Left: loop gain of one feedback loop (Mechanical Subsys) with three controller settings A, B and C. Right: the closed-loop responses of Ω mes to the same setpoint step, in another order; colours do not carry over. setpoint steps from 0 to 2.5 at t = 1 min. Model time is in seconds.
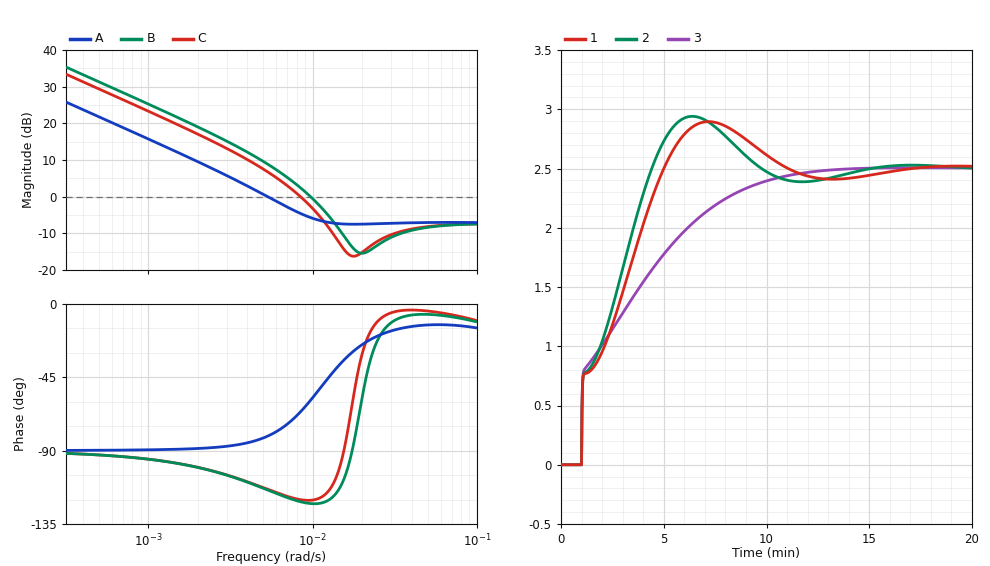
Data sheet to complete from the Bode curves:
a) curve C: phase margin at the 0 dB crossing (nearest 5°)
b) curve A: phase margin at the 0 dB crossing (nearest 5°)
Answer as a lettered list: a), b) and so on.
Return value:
a) 60°
b) 100°
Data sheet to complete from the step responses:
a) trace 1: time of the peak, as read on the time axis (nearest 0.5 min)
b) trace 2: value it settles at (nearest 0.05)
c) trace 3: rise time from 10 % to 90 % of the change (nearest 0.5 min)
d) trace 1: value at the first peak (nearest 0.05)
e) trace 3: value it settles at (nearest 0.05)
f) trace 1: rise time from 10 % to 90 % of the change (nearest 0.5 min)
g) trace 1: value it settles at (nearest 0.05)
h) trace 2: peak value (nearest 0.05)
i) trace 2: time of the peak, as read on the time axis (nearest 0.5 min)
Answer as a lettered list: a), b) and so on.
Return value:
a) 7.0 min
b) 2.50
c) 7.0 min
d) 2.90
e) 2.50
f) 3.5 min
g) 2.50
h) 2.95
i) 6.5 min
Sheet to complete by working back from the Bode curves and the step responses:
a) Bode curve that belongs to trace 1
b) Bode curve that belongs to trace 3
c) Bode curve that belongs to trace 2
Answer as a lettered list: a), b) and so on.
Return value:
a) C
b) A
c) B
